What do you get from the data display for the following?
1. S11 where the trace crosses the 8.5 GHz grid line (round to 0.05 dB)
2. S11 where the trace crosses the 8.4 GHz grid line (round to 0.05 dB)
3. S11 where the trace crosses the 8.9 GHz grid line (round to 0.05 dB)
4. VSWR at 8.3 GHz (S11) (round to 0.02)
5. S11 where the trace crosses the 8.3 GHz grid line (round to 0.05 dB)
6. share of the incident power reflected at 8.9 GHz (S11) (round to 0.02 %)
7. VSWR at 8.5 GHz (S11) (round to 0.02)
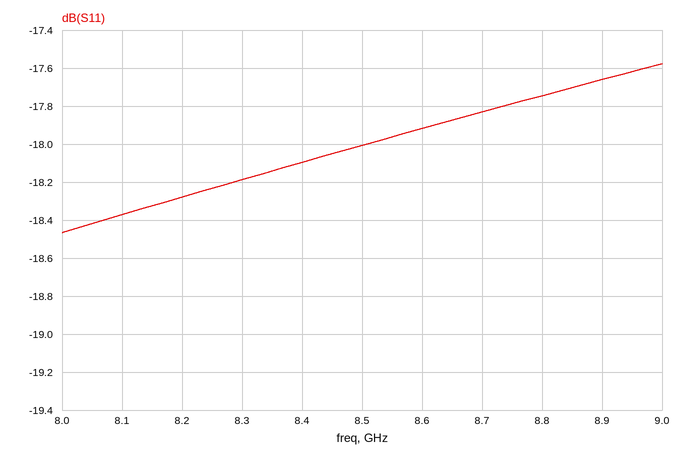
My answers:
-18.00 dB
-18.10 dB
-17.65 dB
1.28
-18.20 dB
1.72 %
1.28
